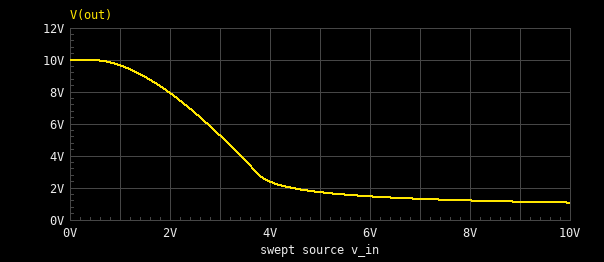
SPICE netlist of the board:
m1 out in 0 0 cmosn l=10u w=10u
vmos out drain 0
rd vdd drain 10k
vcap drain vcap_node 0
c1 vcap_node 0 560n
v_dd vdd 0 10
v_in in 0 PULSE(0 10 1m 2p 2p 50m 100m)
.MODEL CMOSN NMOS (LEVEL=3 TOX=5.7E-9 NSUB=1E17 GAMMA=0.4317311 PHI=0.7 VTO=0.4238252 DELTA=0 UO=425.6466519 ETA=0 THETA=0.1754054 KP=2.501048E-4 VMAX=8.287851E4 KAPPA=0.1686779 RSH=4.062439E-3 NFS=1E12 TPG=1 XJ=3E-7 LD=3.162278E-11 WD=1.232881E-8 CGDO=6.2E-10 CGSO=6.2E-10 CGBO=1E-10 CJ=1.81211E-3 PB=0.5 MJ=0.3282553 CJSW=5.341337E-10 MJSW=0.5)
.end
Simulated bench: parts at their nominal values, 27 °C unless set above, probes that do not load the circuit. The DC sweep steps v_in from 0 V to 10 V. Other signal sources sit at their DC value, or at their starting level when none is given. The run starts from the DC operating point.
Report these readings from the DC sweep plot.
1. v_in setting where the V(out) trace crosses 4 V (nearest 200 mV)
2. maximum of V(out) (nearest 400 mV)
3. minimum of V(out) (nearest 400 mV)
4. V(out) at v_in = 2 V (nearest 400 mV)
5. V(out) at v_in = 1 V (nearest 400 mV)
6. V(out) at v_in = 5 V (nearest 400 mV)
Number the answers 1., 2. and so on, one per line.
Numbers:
1. 3.4 V
2. 10.0 V
3. 1.2 V
4. 8.0 V
5. 9.6 V
6. 1.6 V
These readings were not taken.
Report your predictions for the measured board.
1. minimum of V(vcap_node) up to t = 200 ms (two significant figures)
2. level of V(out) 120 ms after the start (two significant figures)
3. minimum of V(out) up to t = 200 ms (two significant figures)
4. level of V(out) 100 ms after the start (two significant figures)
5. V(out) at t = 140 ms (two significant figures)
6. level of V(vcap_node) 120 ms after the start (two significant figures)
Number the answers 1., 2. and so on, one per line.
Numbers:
1. 1.1 V
2. 1.1 V
3. 1.1 V
4. 10 V
5. 1.1 V
6. 1.1 V
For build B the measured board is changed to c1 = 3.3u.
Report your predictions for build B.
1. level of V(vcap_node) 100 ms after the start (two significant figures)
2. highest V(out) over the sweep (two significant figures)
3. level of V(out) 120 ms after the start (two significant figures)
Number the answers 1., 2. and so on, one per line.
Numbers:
1. 8.0 V
2. 10 V
3. 1.2 V
